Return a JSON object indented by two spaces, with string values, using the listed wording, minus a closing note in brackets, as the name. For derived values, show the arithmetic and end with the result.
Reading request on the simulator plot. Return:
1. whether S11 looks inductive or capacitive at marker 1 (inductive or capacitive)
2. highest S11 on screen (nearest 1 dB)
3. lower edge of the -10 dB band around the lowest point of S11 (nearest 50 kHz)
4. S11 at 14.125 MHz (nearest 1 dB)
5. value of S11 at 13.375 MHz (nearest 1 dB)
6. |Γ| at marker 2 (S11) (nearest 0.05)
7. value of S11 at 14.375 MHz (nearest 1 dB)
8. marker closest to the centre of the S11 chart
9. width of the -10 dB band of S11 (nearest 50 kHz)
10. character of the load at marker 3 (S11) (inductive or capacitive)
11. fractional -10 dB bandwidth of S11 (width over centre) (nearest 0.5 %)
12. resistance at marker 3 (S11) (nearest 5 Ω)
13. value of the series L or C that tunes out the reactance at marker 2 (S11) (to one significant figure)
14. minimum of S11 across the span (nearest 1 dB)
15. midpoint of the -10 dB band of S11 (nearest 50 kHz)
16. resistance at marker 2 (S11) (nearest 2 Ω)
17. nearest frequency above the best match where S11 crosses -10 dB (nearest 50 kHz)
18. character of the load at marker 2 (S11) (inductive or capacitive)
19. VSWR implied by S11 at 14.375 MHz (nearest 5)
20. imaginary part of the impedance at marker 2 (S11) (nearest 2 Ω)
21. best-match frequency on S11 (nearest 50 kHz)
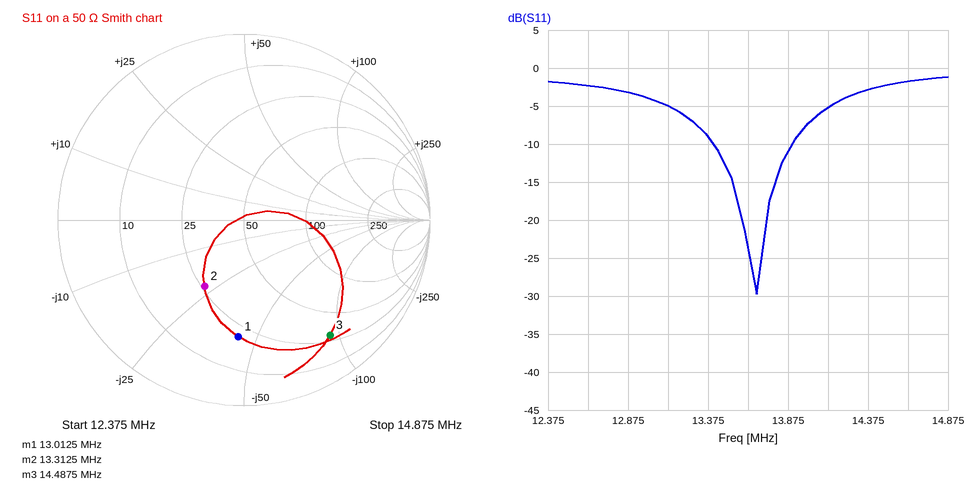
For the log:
{
  "whether S11 looks inductive or capacitive at marker 1": "capacitive",
  "highest S11 on screen": "-1 dB",
  "lower edge of the -10 dB band around the lowest point of S11": "13.40 MHz",
  "S11 at 14.125 MHz": "-5 dB",
  "value of S11 at 13.375 MHz": "-9 dB",
  "|Γ| at marker 2 (S11)": "0.40",
  "value of S11 at 14.375 MHz": "-3 dB",
  "marker closest to the centre of the S11 chart": "marker 2",
  "width of the -10 dB band of S11": "13.90 MHz − 13.40 MHz = 500 kHz",
  "character of the load at marker 3 (S11)": "capacitive",
  "fractional -10 dB bandwidth of S11 (width over centre)": "500 kHz / 13.65 MHz ≈ 3.66 %, so 3.5 % to the nearest 0.5 %",
  "resistance at marker 3 (S11)": "30 Ω",
  "value of the series L or C that tunes out the reactance at marker 2 (S11)": "L = 22 Ω/(2π × 13.3125 MHz) ≈ 263 nH, so 300 nH to one significant figure",
  "minimum of S11 across the span": "-30 dB",
  "midpoint of the -10 dB band of S11": "13.65 MHz",
  "resistance at marker 2 (S11)": "26 Ω",
  "nearest frequency above the best match where S11 crosses -10 dB": "13.90 MHz",
  "character of the load at marker 2 (S11)": "capacitive",
  "VSWR implied by S11 at 14.375 MHz": "|Γ| = 10^(-3/20) = 0.7079; VSWR = (1 + 0.7079)/(1 − 0.7079) ≈ 5.85, so 5 to the nearest 5",
  "imaginary part of the impedance at marker 2 (S11)": "-22 Ω",
  "best-match frequency on S11": "13.70 MHz"
}
